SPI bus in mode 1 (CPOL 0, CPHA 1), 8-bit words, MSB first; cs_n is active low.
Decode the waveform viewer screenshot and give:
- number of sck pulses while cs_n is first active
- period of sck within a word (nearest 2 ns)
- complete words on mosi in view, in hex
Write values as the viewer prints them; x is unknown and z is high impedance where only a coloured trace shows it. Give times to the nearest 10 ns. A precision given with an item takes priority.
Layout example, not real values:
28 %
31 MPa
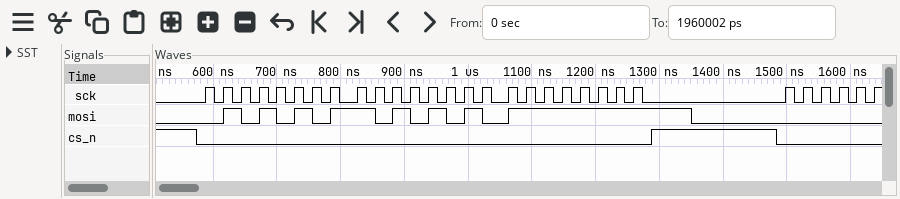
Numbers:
24
28 ns
55, AA, FF
